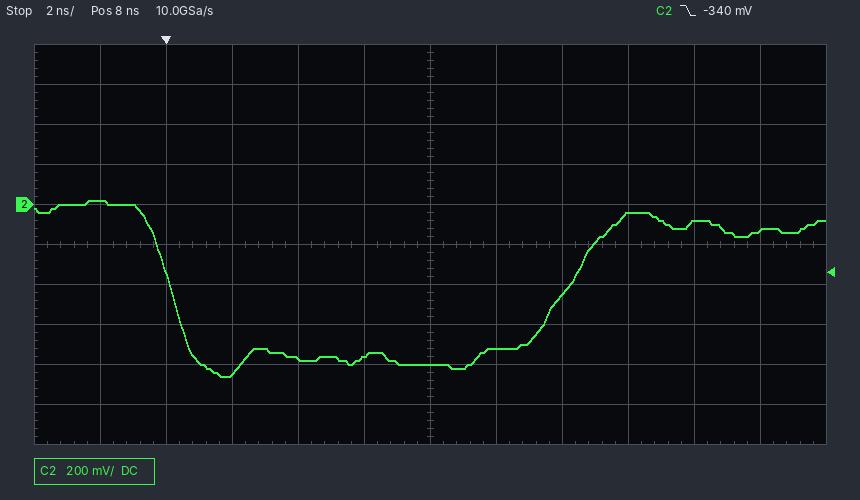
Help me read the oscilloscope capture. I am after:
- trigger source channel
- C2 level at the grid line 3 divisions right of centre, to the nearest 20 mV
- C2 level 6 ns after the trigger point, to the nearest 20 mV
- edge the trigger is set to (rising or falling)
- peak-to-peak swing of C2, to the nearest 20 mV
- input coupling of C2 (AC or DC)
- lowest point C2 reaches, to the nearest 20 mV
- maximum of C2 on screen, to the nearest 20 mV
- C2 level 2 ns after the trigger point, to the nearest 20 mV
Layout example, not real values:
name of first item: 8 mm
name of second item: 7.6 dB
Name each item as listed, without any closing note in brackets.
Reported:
trigger source channel: C2
C2 level at the grid line 3 divisions right of centre, to the nearest 20 mV: -40 mV
C2 level 6 ns after the trigger point, to the nearest 20 mV: -760 mV
edge the trigger is set to: falling
peak-to-peak swing of C2, to the nearest 20 mV: 880 mV
input coupling of C2: DC
lowest point C2 reaches, to the nearest 20 mV: -860 mV
maximum of C2 on screen, to the nearest 20 mV: 20 mV
C2 level 2 ns after the trigger point, to the nearest 20 mV: -840 mV
